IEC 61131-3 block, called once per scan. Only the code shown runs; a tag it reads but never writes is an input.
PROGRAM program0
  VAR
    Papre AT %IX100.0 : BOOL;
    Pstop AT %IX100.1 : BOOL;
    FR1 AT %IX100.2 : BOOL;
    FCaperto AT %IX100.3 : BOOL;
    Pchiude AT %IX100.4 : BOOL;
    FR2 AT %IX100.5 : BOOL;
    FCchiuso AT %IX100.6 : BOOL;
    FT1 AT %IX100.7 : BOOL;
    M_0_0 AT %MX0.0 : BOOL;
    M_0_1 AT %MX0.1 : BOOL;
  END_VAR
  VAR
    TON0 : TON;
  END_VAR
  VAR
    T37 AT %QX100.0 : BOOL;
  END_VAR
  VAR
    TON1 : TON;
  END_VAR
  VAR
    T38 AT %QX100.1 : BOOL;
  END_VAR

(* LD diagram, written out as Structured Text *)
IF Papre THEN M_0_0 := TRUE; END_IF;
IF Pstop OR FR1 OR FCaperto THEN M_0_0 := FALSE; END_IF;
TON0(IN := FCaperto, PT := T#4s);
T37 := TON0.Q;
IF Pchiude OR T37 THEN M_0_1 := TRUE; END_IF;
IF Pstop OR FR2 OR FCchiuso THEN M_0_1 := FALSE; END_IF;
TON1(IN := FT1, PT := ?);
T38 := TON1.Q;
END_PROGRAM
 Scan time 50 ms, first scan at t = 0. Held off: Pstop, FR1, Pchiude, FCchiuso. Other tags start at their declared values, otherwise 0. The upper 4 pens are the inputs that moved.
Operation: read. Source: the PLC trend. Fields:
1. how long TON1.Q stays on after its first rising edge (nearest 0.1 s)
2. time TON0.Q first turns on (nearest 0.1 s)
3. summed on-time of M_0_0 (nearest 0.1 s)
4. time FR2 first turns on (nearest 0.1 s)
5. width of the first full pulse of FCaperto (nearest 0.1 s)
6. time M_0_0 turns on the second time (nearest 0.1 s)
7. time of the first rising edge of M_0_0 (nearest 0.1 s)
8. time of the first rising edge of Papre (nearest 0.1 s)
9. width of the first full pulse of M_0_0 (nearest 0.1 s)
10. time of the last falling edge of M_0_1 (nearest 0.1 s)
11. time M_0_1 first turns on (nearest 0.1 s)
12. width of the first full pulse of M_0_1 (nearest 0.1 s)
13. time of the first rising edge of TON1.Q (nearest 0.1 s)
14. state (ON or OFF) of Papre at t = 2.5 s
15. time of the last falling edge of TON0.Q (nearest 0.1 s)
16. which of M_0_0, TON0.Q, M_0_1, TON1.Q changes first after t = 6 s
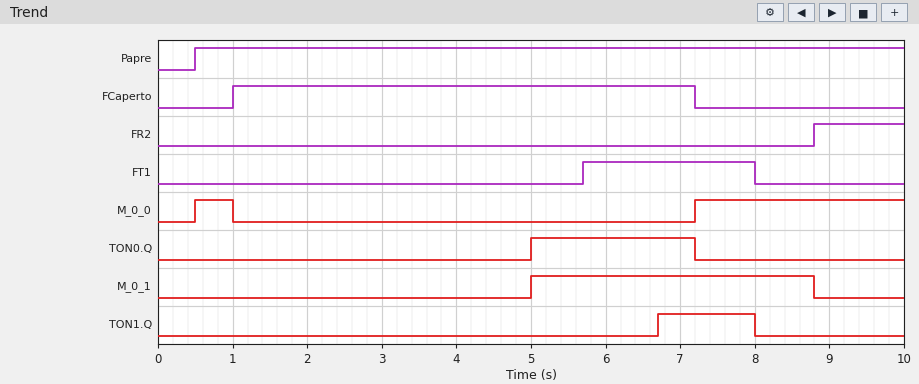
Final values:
1.3 s
5.0 s
3.3 s
8.8 s
6.2 s
7.2 s
0.5 s
0.5 s
0.5 s
8.8 s
5.0 s
3.8 s
6.7 s
ON
7.2 s
TON1.Q
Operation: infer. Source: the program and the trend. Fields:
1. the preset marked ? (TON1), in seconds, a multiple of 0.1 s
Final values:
1.0 s
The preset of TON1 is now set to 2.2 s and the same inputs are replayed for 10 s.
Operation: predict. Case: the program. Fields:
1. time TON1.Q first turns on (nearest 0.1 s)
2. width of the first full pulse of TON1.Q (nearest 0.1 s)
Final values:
7.9 s
0.1 s
